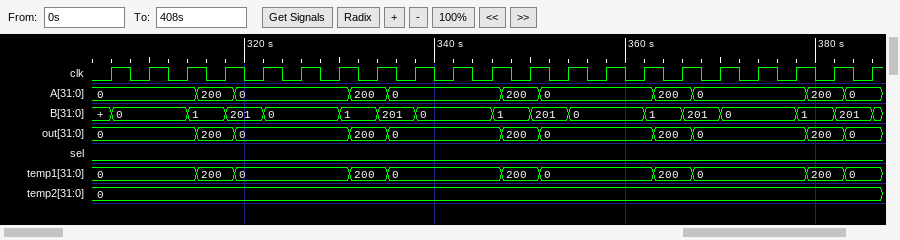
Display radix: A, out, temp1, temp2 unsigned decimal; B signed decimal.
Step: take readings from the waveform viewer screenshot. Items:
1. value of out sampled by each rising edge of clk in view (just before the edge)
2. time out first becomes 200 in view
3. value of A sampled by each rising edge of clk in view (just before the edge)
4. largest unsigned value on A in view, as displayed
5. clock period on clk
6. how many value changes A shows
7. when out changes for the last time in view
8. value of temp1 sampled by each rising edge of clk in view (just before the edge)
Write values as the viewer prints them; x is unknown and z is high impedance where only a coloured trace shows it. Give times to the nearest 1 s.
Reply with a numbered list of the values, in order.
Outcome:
1. 0, 0, 0, 200, 0, 0, 0, 200, 0, 0, 0, 200, 0, 0, 0, 200, 0, 0, 0, 200, 0
2. 315 s
3. 0, 0, 0, 200, 0, 0, 0, 200, 0, 0, 0, 200, 0, 0, 0, 200, 0, 0, 0, 200, 0
4. 200
5. 4 s
6. 10
7. 383 s
8. 0, 0, 0, 200, 0, 0, 0, 200, 0, 0, 0, 200, 0, 0, 0, 200, 0, 0, 0, 200, 0
